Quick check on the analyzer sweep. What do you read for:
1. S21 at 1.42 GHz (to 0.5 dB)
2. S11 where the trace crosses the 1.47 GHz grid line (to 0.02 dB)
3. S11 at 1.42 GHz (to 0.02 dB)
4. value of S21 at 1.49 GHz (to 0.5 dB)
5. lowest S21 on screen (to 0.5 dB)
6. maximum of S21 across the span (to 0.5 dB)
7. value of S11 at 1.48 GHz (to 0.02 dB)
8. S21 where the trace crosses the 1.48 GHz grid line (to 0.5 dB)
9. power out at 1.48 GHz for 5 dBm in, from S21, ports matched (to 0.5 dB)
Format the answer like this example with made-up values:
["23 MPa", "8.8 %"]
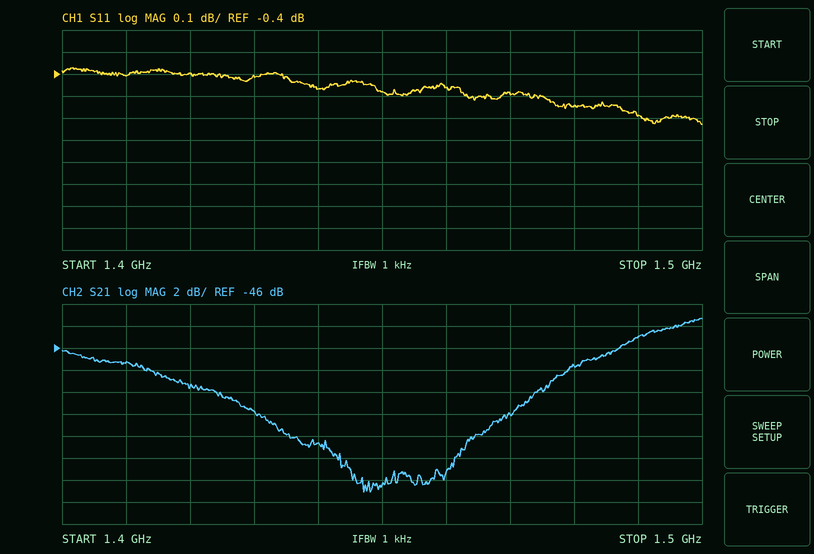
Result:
["-49.5 dB", "-0.48 dB", "-0.40 dB", "-45.0 dB", "-59.0 dB", "-43.5 dB", "-0.54 dB", "-47.5 dB", "-42.5 dBm"]
